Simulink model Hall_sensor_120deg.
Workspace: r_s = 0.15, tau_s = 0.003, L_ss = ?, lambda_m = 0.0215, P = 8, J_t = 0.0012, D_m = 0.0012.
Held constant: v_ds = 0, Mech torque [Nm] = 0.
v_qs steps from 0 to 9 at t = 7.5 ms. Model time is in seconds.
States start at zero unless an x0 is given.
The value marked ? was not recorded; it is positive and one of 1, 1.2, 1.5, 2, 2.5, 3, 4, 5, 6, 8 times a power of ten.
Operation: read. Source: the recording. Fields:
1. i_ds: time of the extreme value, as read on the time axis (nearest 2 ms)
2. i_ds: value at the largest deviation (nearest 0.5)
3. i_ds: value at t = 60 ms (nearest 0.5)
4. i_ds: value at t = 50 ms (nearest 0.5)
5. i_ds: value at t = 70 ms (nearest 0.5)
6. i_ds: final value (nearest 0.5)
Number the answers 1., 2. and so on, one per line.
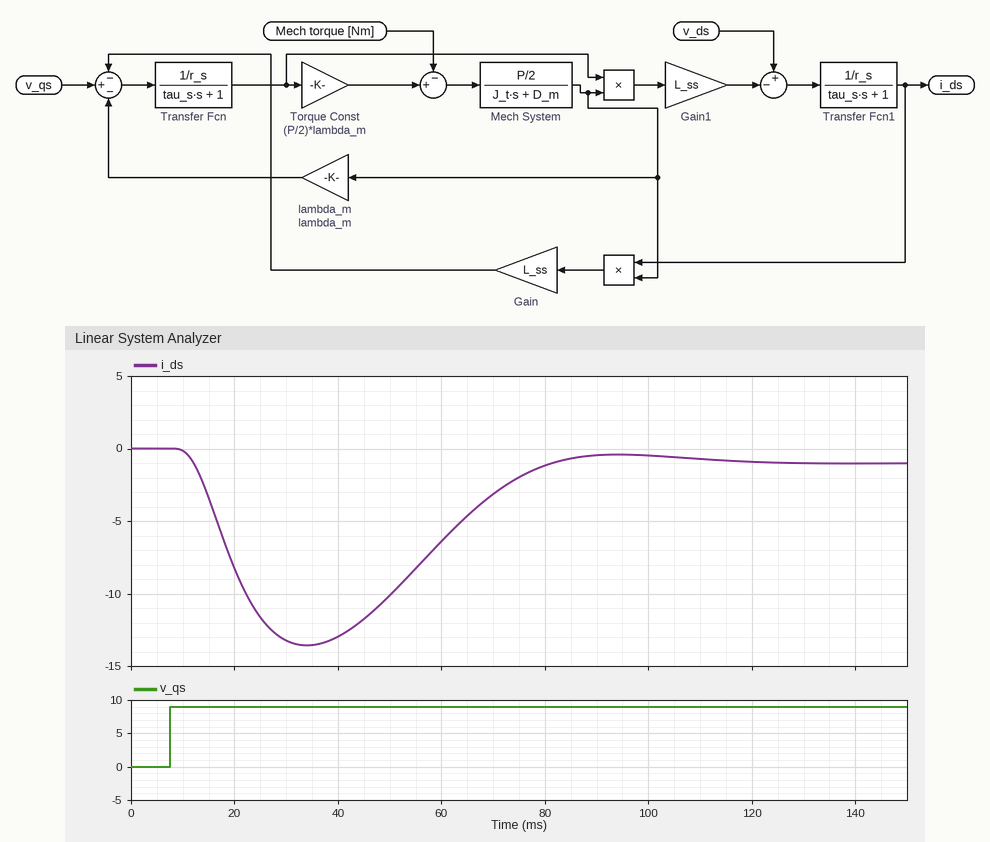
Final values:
1. 34 ms
2. -13.5
3. -6.5
4. -10.0
5. -3.0
6. -1.0
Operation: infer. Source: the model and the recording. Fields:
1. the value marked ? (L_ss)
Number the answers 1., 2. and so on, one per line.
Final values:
1. 0.00025
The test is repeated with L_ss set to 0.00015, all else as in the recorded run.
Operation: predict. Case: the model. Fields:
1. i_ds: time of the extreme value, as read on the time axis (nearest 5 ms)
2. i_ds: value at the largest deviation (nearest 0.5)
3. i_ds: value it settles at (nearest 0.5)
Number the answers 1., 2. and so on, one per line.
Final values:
1. 30 ms
2. -7.5
3. -0.5
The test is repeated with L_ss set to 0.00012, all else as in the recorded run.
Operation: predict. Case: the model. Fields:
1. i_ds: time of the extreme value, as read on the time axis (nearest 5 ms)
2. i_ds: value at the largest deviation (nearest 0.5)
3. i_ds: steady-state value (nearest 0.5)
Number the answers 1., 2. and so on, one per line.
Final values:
1. 30 ms
2. -6.0
3. -0.5
